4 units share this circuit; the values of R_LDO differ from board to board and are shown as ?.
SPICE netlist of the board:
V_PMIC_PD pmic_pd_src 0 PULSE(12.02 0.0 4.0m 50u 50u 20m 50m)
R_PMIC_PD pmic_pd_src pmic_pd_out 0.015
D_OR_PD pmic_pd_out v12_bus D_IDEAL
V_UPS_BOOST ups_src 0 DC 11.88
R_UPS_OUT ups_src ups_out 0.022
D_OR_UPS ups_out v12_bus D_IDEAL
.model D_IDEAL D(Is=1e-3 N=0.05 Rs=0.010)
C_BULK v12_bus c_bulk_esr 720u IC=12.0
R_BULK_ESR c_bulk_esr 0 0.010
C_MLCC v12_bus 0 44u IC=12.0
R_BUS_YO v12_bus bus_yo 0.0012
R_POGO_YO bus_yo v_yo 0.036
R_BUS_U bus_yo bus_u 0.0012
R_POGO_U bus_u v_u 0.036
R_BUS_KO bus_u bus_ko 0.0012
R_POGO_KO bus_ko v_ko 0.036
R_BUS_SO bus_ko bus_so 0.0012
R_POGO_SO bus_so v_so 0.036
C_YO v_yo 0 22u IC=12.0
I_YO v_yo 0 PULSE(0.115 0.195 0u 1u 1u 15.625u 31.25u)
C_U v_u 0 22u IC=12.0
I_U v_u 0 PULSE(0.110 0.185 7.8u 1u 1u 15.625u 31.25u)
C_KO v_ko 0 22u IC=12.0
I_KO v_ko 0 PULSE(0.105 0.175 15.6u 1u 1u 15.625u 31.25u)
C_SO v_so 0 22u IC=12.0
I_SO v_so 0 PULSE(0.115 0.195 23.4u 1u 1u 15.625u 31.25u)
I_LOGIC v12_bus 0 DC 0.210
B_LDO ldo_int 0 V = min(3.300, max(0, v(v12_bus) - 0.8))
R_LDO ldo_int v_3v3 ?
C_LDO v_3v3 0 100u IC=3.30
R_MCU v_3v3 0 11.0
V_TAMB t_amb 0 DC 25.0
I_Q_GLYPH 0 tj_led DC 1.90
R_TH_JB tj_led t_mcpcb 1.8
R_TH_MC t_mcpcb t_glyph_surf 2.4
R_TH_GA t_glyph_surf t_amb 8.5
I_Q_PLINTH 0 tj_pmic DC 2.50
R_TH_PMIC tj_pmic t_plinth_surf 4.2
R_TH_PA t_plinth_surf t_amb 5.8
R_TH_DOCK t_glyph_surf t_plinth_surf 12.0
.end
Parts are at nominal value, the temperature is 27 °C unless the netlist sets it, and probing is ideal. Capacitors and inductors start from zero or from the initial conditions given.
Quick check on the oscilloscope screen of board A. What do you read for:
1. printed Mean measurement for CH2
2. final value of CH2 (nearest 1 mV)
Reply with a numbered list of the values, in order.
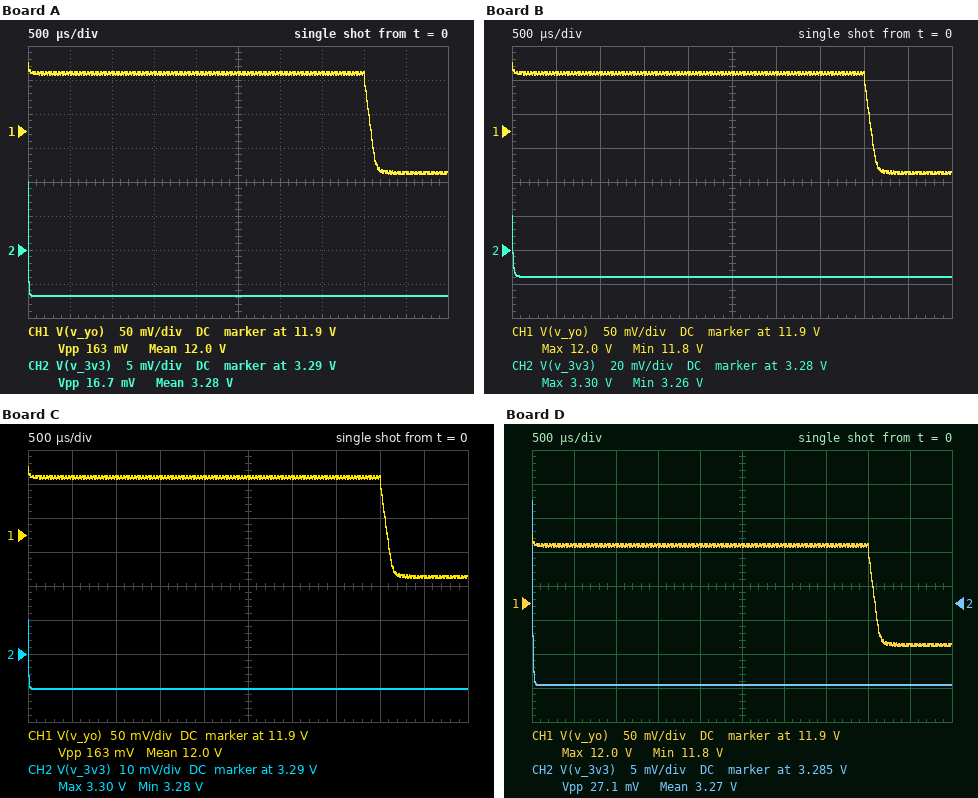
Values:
1. 3.28 V
2. 3.283 V
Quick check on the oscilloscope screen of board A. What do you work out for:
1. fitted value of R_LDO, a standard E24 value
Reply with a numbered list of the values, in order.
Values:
1. 0.056 Ω
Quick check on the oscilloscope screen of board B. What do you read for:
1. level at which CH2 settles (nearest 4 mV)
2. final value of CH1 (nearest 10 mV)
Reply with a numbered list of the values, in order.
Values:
1. 3.264 V
2. 11.84 V
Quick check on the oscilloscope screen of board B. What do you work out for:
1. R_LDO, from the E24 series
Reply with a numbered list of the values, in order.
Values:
1. 0.12 Ω
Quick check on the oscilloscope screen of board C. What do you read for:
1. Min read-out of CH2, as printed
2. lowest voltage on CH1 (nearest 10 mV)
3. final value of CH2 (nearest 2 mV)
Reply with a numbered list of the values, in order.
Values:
1. 3.28 V
2. 11.84 V
3. 3.280 V
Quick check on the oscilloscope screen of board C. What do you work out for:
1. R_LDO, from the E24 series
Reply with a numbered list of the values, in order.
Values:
1. 0.068 Ω
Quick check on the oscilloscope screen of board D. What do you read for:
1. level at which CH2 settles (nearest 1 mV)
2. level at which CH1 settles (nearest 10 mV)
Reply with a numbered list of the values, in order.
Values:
1. 3.273 V
2. 11.84 V
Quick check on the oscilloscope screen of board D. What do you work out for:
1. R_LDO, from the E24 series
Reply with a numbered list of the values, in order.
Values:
1. 0.091 Ω
